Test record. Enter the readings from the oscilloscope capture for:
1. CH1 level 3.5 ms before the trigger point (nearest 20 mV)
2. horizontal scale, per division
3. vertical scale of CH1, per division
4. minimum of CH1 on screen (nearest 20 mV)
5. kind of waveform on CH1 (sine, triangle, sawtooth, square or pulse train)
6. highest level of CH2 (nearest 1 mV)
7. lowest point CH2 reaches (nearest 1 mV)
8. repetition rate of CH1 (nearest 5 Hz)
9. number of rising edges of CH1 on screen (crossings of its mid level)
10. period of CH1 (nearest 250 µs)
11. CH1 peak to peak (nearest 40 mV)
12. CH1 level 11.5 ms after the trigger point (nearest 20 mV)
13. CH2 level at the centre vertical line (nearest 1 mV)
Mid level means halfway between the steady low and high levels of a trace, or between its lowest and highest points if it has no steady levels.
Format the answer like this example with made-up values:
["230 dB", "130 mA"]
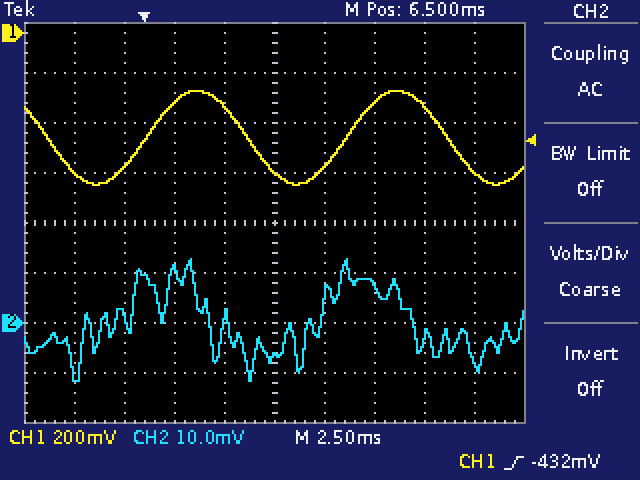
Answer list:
["-560 mV", "2.5 ms", "200 mV", "-600 mV", "sine", "13 mV", "-12 mV", "100 Hz", "2", "10.00 ms", "360 mV", "-280 mV", "-7 mV"]
